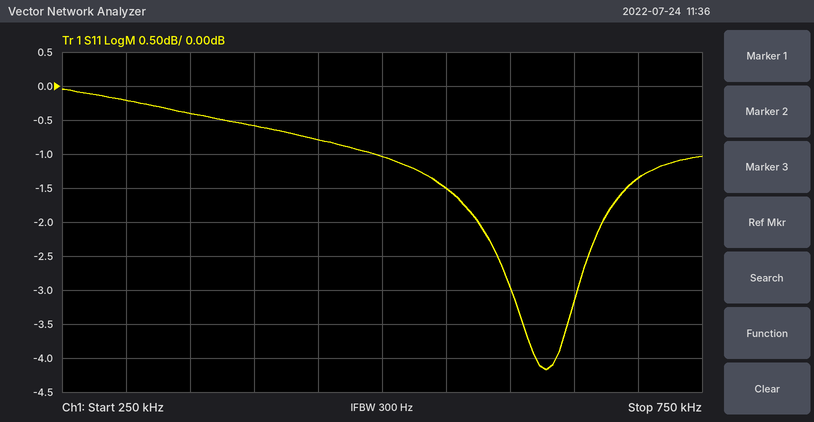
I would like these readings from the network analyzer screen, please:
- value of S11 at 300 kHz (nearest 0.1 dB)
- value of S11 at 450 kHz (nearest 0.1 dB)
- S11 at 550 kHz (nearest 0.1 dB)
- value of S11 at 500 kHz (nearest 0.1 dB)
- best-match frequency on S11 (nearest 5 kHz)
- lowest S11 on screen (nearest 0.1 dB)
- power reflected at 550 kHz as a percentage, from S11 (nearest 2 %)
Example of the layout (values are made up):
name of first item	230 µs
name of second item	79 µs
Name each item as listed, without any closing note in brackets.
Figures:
value of S11 at 300 kHz	-0.2 dB
value of S11 at 450 kHz	-0.8 dB
S11 at 550 kHz	-1.5 dB
value of S11 at 500 kHz	-1.0 dB
best-match frequency on S11	630 kHz
lowest S11 on screen	-4.2 dB
power reflected at 550 kHz as a percentage, from S11	70 %
